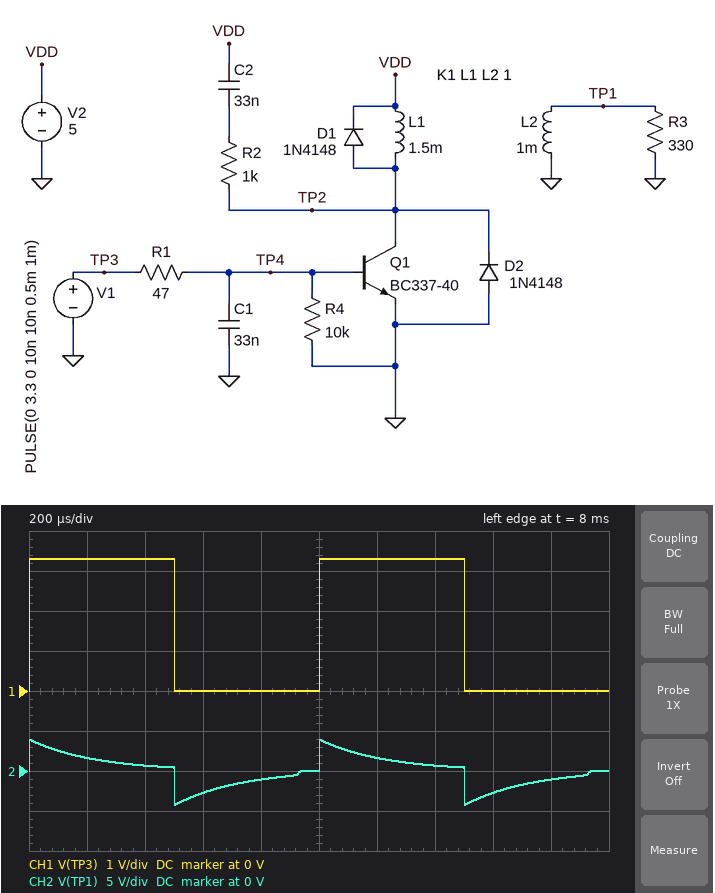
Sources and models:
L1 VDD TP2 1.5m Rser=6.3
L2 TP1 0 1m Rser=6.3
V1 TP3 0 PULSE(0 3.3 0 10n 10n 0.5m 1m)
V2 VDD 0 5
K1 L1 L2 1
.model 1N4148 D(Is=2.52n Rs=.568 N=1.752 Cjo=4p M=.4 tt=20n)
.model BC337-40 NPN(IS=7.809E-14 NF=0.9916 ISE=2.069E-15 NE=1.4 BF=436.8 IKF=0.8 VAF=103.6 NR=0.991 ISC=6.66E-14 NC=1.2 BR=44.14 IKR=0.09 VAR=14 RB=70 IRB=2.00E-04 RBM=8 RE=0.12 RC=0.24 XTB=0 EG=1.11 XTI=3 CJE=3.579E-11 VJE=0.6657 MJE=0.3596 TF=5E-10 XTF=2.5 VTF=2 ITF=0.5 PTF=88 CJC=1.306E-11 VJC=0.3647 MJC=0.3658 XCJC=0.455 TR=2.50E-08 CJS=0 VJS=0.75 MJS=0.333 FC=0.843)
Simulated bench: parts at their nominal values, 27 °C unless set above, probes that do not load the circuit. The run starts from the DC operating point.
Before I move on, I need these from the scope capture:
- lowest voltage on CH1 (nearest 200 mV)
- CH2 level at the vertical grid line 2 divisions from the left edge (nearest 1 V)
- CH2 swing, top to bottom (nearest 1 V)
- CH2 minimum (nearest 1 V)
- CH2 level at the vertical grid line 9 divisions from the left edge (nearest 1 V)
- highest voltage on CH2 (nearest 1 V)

0 V
1 V
8 V
-4 V
-1 V
4 V
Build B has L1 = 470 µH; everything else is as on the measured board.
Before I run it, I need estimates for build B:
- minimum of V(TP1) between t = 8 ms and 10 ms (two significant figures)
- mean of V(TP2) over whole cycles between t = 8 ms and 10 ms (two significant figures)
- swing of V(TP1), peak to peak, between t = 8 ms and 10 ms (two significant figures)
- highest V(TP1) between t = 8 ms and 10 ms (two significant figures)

-8.2 V
2.8 V
15 V
6.8 V
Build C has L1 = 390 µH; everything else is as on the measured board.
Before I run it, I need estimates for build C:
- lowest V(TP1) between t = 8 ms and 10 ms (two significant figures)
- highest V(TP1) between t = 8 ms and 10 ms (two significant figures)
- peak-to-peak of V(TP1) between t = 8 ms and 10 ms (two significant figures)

-8.9 V
7.4 V
16 V
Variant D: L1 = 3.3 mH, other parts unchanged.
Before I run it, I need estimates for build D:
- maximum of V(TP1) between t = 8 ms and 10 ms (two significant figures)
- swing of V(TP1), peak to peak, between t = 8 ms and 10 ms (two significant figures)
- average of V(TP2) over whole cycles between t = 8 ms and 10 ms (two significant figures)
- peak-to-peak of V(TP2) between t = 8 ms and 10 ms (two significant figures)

2.3 V
4.6 V
3.1 V
6.1 V
